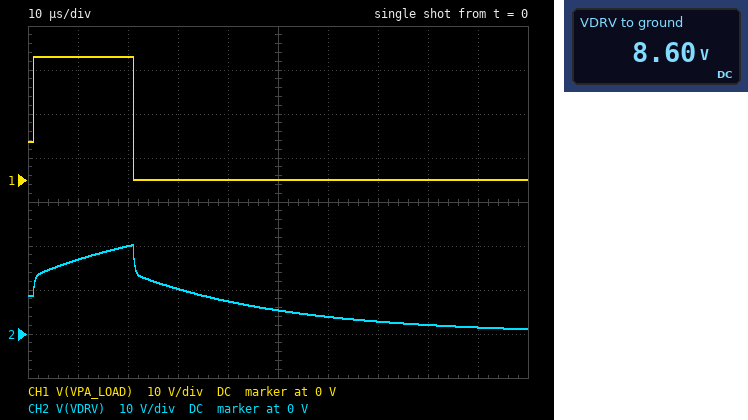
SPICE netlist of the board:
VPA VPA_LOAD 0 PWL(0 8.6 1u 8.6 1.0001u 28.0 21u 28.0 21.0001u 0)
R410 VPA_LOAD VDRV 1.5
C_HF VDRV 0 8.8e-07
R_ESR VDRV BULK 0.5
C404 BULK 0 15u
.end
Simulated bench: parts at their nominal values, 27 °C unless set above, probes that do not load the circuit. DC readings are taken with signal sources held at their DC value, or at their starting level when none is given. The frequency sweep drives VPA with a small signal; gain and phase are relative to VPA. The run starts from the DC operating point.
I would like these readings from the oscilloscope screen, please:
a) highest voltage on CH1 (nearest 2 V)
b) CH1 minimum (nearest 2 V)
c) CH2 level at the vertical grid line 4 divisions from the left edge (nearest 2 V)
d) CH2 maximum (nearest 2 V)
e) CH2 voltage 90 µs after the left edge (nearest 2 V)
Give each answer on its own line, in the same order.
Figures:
28 V
0 V
8 V
20 V
2 V
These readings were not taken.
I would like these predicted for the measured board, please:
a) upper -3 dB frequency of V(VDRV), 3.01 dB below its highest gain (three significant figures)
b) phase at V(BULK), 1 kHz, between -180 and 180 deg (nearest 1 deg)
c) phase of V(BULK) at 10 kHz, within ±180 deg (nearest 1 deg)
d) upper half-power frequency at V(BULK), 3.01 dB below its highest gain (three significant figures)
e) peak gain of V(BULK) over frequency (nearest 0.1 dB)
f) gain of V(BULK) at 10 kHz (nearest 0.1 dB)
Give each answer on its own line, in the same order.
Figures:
5.46 kHz
-11 deg
-64 deg
5.13 kHz
0 dB
-6.8 dB
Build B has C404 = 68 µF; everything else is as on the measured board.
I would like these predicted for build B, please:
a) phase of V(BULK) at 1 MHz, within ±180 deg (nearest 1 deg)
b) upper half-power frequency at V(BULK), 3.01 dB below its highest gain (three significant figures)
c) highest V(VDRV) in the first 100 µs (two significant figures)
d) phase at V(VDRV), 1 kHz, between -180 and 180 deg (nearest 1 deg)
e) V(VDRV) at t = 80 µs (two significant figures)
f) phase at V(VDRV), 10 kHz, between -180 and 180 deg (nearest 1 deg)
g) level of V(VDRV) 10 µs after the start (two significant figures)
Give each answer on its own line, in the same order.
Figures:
-154 deg
1.16 kHz
15 V
-29 deg
5.5 V
-20 deg
14 V
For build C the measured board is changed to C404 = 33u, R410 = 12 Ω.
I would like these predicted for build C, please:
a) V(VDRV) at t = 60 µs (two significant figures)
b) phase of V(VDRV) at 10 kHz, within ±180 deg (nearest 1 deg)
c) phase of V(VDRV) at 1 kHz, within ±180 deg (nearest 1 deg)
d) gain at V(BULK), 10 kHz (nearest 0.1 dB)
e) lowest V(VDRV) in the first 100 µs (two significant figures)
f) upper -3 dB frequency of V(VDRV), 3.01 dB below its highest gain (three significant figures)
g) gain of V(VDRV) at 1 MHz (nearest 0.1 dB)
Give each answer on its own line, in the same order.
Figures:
8.3 V
-43 deg
-64 deg
-28.5 dB
7.6 V
377 Hz
-37.0 dB
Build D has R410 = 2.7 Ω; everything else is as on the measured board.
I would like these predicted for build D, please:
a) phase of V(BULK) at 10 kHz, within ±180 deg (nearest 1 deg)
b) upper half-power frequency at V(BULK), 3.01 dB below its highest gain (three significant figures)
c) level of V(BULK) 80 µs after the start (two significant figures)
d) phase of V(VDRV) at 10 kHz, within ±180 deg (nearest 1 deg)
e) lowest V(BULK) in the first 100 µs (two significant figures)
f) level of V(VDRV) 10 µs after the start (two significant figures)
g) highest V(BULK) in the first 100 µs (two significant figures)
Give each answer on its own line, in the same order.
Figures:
-74 deg
3.18 kHz
4.6 V
-48 deg
3.1 V
14 V
15 V
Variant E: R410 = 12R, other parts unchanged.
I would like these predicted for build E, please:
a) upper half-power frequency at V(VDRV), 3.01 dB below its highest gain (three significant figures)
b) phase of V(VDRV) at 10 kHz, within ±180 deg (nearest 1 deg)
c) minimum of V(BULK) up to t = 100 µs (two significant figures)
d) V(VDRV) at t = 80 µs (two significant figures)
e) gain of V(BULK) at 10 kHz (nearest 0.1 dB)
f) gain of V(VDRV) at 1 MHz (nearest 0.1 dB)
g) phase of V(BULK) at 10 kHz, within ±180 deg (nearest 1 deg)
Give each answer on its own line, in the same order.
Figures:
806 Hz
-62 deg
7.0 V
7.5 V
-21.9 dB
-37.1 dB
-87 deg
